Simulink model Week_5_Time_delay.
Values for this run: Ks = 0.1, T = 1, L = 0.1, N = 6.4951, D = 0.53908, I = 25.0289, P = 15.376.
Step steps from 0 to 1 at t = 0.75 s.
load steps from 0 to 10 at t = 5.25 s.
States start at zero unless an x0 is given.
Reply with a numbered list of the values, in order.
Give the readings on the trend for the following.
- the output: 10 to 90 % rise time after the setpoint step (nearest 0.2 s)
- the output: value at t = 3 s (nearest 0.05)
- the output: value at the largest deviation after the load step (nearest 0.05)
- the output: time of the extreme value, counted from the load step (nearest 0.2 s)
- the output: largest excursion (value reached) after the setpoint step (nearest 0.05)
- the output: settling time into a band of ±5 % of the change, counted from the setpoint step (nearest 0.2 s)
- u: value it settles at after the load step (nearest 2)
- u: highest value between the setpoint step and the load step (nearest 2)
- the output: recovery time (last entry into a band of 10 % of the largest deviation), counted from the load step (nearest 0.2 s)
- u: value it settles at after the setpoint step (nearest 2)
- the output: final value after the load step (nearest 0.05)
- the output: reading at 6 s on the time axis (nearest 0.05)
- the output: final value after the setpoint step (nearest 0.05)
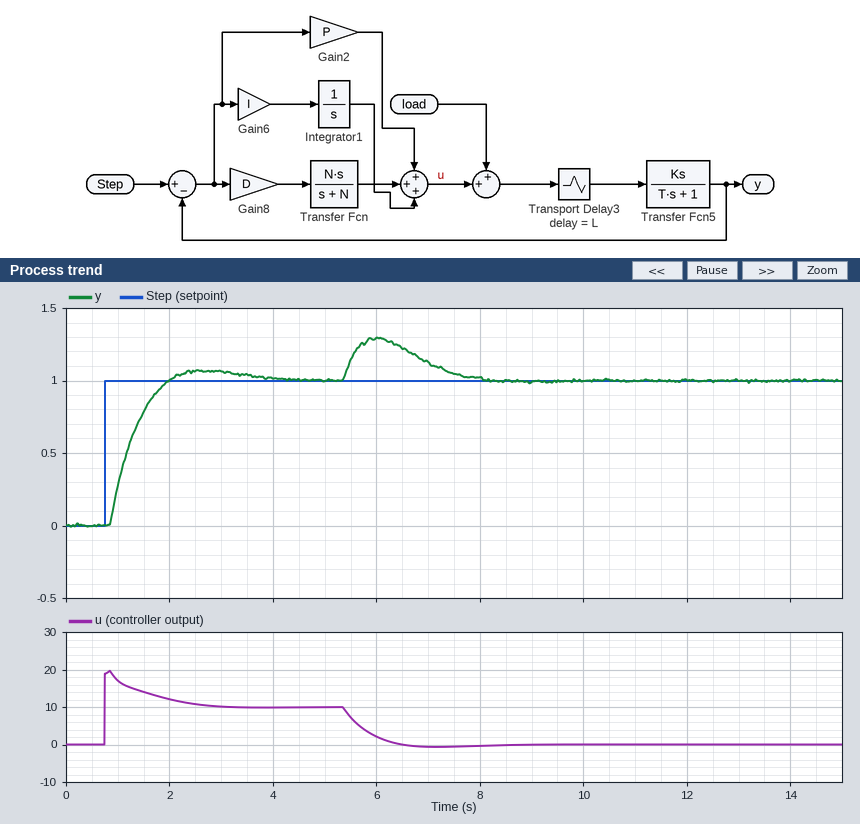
1. 0.8 s
2. 1.05
3. 1.30
4. 0.8 s
5. 1.05
6. 2.4 s
7. 0
8. 20
9. 2.4 s
10. 10
11. 1.00
12. 1.30
13. 1.00
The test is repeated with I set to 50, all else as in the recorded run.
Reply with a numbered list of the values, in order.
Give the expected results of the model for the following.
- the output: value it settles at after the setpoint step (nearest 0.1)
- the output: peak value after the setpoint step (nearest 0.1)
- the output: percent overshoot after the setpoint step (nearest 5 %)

1. 1.0
2. 1.2
3. 25 %
